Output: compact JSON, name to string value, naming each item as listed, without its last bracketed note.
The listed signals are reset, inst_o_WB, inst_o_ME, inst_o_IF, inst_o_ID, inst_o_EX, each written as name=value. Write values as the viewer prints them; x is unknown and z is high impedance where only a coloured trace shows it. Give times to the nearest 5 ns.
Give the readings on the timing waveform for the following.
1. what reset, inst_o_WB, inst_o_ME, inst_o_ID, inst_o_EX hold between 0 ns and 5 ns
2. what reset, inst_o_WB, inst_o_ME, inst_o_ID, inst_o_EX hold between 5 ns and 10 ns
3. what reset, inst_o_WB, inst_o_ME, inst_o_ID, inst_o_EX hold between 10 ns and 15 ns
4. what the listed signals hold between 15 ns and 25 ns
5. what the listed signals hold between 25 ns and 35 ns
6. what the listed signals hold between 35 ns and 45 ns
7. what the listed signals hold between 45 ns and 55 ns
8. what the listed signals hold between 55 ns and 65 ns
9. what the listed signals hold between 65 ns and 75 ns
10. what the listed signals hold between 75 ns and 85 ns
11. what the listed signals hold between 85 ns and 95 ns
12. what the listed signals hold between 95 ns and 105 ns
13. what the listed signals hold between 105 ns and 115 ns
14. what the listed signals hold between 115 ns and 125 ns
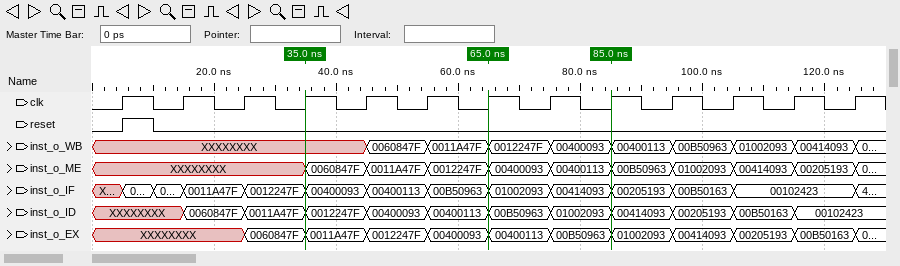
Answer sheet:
{"what reset, inst_o_WB, inst_o_ME, inst_o_ID, inst_o_EX hold between 0 ns and 5 ns": "reset=0, inst_o_WB=XXXXXXXX, inst_o_ME=XXXXXXXX, inst_o_ID=XXXXXXXX, inst_o_EX=XXXXXXXX", "what reset, inst_o_WB, inst_o_ME, inst_o_ID, inst_o_EX hold between 5 ns and 10 ns": "reset=1, inst_o_WB=XXXXXXXX, inst_o_ME=XXXXXXXX, inst_o_ID=XXXXXXXX, inst_o_EX=XXXXXXXX", "what reset, inst_o_WB, inst_o_ME, inst_o_ID, inst_o_EX hold between 10 ns and 15 ns": "reset=0, inst_o_WB=XXXXXXXX, inst_o_ME=XXXXXXXX, inst_o_ID=XXXXXXXX, inst_o_EX=XXXXXXXX", "what the listed signals hold between 15 ns and 25 ns": "reset=0, inst_o_WB=XXXXXXXX, inst_o_ME=XXXXXXXX, inst_o_IF=0011A47F, inst_o_ID=0060847F, inst_o_EX=XXXXXXXX", "what the listed signals hold between 25 ns and 35 ns": "reset=0, inst_o_WB=XXXXXXXX, inst_o_ME=XXXXXXXX, inst_o_IF=0012247F, inst_o_ID=0011A47F, inst_o_EX=0060847F", "what the listed signals hold between 35 ns and 45 ns": "reset=0, inst_o_WB=XXXXXXXX, inst_o_ME=0060847F, inst_o_IF=00400093, inst_o_ID=0012247F, inst_o_EX=0011A47F", "what the listed signals hold between 45 ns and 55 ns": "reset=0, inst_o_WB=0060847F, inst_o_ME=0011A47F, inst_o_IF=00400113, inst_o_ID=00400093, inst_o_EX=0012247F", "what the listed signals hold between 55 ns and 65 ns": "reset=0, inst_o_WB=0011A47F, inst_o_ME=0012247F, inst_o_IF=00B50963, inst_o_ID=00400113, inst_o_EX=00400093", "what the listed signals hold between 65 ns and 75 ns": "reset=0, inst_o_WB=0012247F, inst_o_ME=00400093, inst_o_IF=01002093, inst_o_ID=00B50963, inst_o_EX=00400113", "what the listed signals hold between 75 ns and 85 ns": "reset=0, inst_o_WB=00400093, inst_o_ME=00400113, inst_o_IF=00414093, inst_o_ID=01002093, inst_o_EX=00B50963", "what the listed signals hold between 85 ns and 95 ns": "reset=0, inst_o_WB=00400113, inst_o_ME=00B50963, inst_o_IF=00205193, inst_o_ID=00414093, inst_o_EX=01002093", "what the listed signals hold between 95 ns and 105 ns": "reset=0, inst_o_WB=00B50963, inst_o_ME=01002093, inst_o_IF=00B50163, inst_o_ID=00205193, inst_o_EX=00414093", "what the listed signals hold between 105 ns and 115 ns": "reset=0, inst_o_WB=01002093, inst_o_ME=00414093, inst_o_IF=00102423, inst_o_ID=00B50163, inst_o_EX=00205193", "what the listed signals hold between 115 ns and 125 ns": "reset=0, inst_o_WB=00414093, inst_o_ME=00205193, inst_o_IF=00102423, inst_o_ID=00102423, inst_o_EX=00B50163"}
